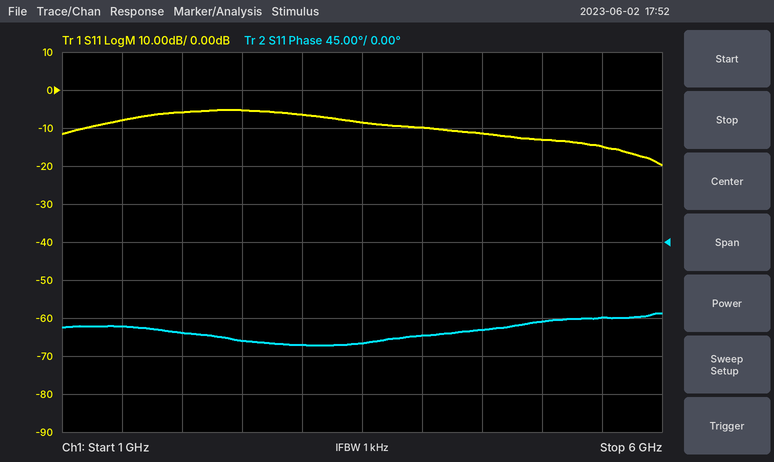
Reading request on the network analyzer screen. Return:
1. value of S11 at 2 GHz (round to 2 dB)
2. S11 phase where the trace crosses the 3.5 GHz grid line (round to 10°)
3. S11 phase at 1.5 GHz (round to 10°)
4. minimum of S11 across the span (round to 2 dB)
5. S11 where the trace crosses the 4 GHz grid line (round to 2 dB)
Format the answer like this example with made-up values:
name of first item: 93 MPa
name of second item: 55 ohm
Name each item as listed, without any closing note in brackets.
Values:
value of S11 at 2 GHz: -6 dB
S11 phase where the trace crosses the 3.5 GHz grid line: -120°
S11 phase at 1.5 GHz: -100°
minimum of S11 across the span: -20 dB
S11 where the trace crosses the 4 GHz grid line: -10 dB
